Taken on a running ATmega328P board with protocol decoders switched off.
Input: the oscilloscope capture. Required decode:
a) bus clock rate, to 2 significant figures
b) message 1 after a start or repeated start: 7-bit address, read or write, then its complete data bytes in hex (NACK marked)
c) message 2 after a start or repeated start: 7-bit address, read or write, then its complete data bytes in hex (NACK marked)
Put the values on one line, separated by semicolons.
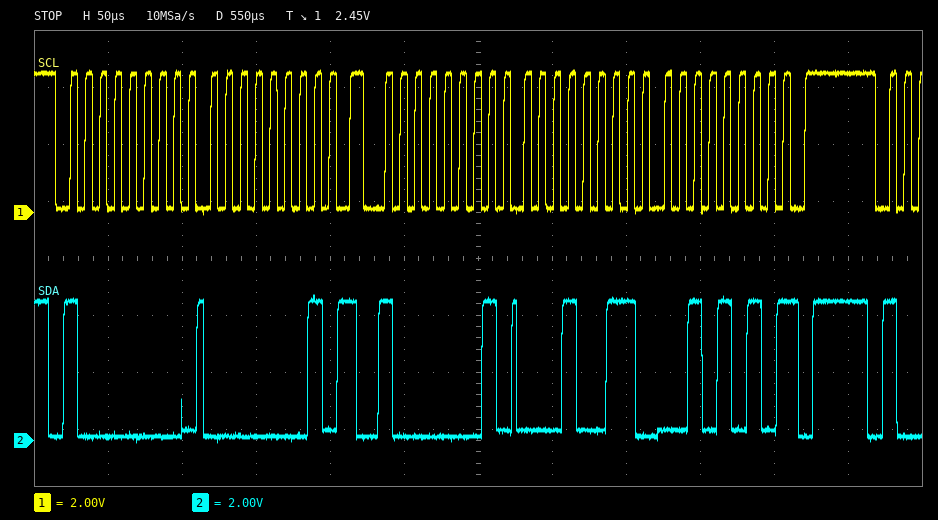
100 kHz; 0x40 write: 01; 0x40 read: 13 2A NACK
